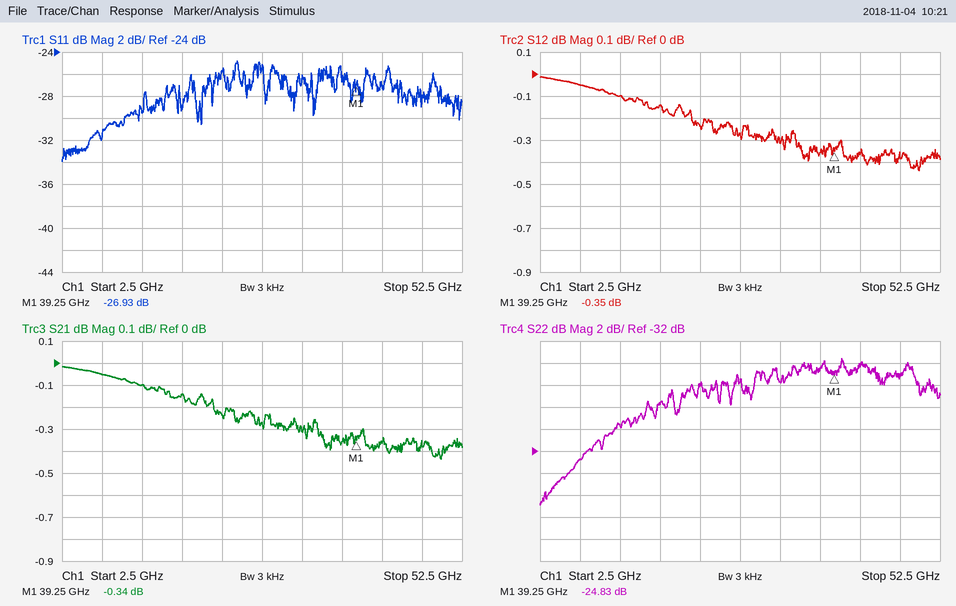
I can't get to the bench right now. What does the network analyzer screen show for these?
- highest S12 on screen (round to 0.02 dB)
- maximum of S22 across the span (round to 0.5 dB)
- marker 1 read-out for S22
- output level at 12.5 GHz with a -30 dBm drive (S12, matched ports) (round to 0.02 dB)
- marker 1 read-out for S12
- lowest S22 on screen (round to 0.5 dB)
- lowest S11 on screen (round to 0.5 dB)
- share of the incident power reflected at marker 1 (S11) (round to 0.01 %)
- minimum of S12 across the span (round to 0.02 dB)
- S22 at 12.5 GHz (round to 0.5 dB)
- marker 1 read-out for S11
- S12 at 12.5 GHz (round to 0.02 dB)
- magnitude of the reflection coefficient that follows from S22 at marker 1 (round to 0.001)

-0.02 dB
-23.5 dB
-24.83 dB
-30.10 dBm
-0.35 dB
-37.0 dB
-34.0 dB
0.20 %
-0.44 dB
-29.5 dB
-26.93 dB
-0.10 dB
0.057
